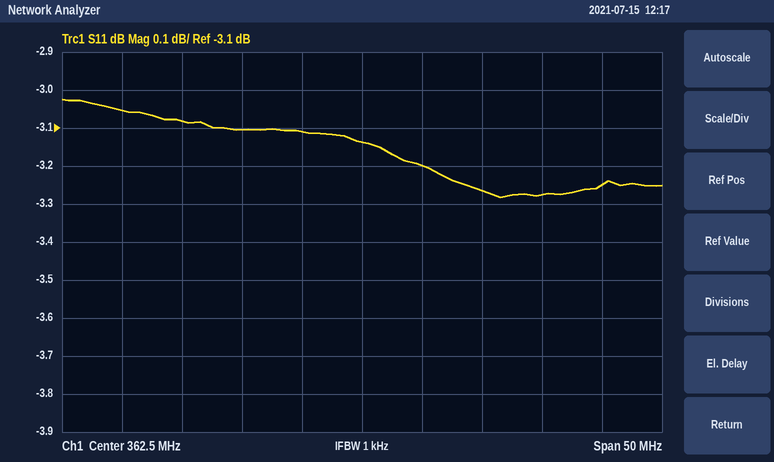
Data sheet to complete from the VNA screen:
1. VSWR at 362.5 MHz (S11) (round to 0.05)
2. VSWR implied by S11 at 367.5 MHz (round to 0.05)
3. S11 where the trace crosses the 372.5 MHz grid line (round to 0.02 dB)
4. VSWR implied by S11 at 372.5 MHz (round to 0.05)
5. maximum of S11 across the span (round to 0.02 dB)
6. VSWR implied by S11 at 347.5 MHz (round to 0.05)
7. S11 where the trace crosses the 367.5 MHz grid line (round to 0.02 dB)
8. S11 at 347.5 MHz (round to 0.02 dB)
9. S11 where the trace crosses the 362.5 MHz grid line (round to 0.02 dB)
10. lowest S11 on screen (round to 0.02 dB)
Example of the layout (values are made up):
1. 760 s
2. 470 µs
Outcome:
1. 5.60
2. 5.50
3. -3.26 dB
4. 5.40
5. -3.02 dB
6. 5.70
7. -3.20 dB
8. -3.08 dB
9. -3.14 dB
10. -3.28 dB
